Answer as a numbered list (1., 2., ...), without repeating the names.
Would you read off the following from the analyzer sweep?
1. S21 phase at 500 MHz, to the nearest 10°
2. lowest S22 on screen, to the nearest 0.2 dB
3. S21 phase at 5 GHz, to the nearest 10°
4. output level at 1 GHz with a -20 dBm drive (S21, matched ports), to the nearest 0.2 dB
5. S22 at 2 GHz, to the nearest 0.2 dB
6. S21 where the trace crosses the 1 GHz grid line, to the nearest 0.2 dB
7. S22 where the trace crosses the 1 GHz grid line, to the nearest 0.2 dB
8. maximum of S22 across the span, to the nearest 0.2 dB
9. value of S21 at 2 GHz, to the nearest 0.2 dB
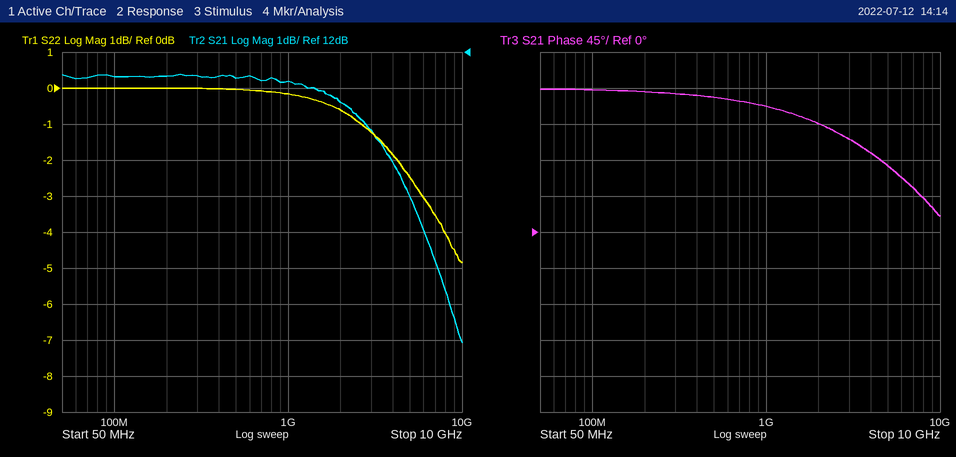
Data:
1. 170°
2. -4.8 dB
3. 80°
4. -8.8 dBm
5. -0.6 dB
6. 11.2 dB
7. -0.2 dB
8. 0.0 dB
9. 10.6 dB
